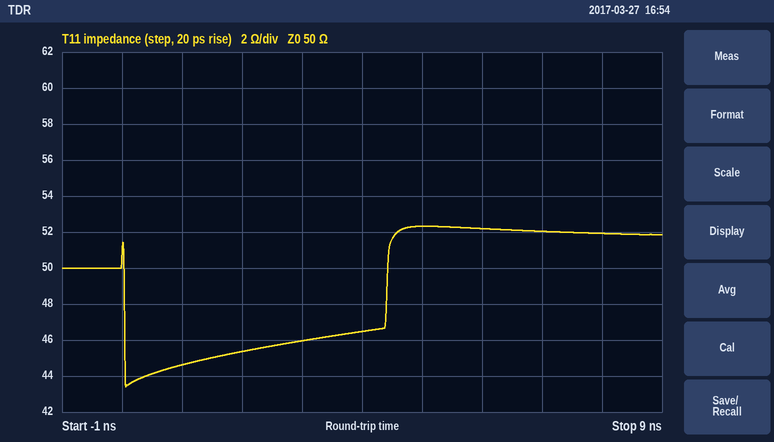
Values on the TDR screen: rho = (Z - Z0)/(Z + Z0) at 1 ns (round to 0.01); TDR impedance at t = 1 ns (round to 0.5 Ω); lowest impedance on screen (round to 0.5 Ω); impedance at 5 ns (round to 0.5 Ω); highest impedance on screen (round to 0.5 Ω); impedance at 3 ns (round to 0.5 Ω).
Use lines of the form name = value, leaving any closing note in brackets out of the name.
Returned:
rho = (Z - Z0)/(Z + Z0) at 1 ns = -0.06
TDR impedance at t = 1 ns = 44.5 Ω
lowest impedance on screen = 43.5 Ω
impedance at 5 ns = 52.5 Ω
highest impedance on screen = 52.5 Ω
impedance at 3 ns = 46.0 Ω
